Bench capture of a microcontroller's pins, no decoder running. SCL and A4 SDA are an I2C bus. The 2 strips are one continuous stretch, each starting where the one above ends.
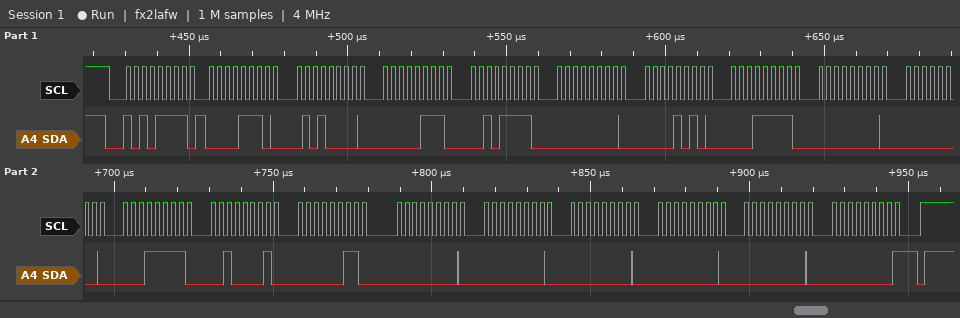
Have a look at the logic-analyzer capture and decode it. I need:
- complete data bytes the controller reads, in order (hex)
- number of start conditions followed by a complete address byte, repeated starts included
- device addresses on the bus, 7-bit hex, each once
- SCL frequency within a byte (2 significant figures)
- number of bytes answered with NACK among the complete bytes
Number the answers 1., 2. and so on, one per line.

1. 0E 50 07 2F 00 0A 1F 00 00 1F 21 03 00 00 00 00 00 00
2. 1
3. 0x57
4. 400 kHz
5. 1
